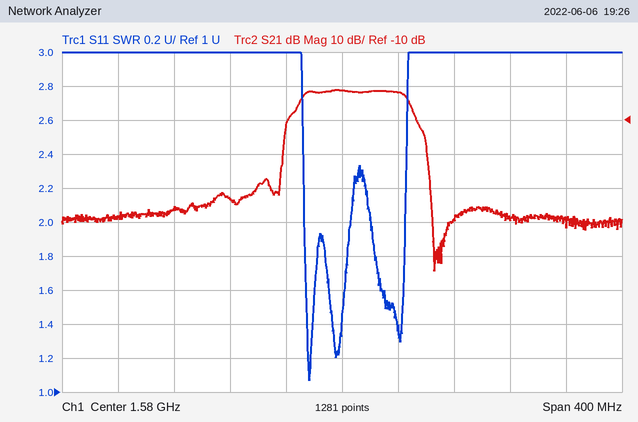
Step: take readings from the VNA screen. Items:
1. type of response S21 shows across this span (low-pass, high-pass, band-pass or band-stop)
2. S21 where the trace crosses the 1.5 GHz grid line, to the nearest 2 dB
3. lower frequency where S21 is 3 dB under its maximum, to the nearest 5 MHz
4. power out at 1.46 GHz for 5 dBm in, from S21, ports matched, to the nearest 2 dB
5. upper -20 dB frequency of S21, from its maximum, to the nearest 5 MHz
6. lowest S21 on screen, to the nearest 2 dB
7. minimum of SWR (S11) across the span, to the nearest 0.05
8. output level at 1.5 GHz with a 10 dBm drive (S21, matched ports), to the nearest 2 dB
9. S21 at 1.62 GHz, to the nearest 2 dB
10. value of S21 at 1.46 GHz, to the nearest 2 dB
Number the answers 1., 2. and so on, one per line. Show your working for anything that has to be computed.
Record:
1. band-pass
2. -34 dB
3. 1.550 GHz
4. 5 dBm + (-36 dB) = -32 dBm
5. 1.640 GHz
6. -54 dB
7. 1.05
8. 10 dBm + (-34 dB) = -24 dBm
9. -2 dB
10. -36 dB
